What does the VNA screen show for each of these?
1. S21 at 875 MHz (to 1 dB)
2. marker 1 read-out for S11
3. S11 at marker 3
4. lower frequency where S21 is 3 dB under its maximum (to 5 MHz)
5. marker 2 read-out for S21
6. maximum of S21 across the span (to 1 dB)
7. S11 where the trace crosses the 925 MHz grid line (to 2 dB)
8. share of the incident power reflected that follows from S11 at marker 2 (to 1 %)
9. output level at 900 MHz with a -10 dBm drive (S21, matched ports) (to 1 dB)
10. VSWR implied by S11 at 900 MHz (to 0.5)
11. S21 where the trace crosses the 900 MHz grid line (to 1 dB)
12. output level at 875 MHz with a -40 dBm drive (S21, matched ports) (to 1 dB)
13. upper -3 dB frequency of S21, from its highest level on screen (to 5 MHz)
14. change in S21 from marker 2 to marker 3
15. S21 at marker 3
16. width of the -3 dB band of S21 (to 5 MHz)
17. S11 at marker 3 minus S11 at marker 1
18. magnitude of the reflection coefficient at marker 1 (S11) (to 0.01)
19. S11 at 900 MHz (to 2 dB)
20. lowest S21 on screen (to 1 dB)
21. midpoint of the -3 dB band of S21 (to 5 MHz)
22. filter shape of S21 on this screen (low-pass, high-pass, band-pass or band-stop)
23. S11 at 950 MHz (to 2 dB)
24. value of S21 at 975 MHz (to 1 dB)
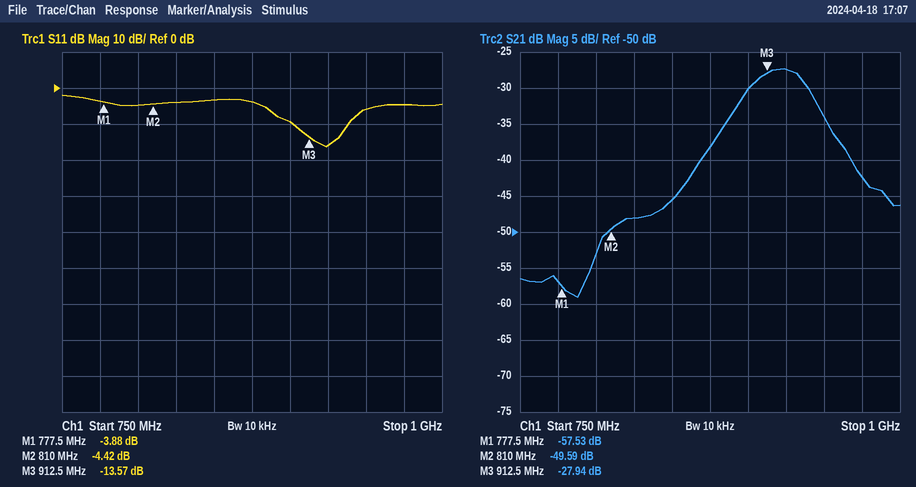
-38 dB
-3.88 dB
-13.57 dB
900 MHz
-49.59 dB
-27 dB
-16 dB
36 %
-40 dBm
2.0
-30 dB
-78 dBm
940 MHz
21.65 dB
-27.94 dB
40 MHz
-9.69 dB
0.64
-10 dB
-59 dB
920 MHz
band-pass
-6 dB
-42 dB
